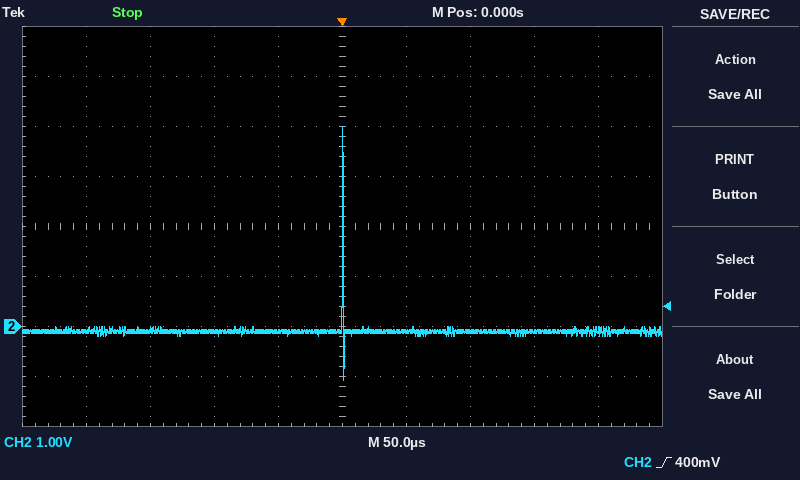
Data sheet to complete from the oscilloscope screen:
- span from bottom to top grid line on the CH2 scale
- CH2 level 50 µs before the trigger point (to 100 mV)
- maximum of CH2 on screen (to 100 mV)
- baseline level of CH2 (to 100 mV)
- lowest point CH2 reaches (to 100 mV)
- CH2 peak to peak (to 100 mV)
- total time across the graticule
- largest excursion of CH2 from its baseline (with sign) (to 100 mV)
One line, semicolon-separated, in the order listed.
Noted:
8 V; -100 mV; 4.0 V; -100 mV; -1.1 V; 5.1 V; 500 µs; +4.1 V
